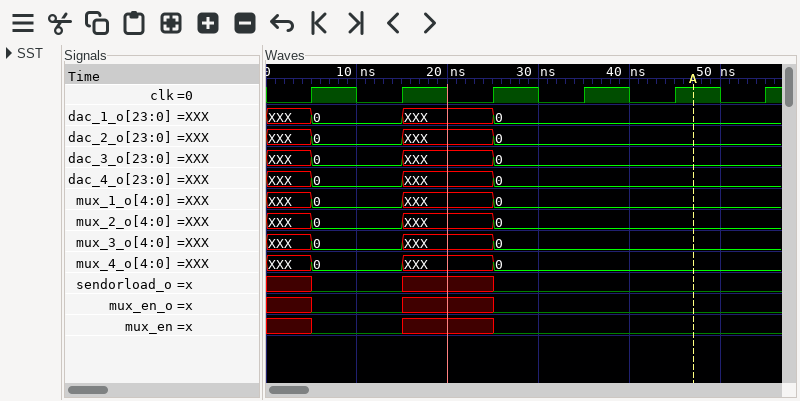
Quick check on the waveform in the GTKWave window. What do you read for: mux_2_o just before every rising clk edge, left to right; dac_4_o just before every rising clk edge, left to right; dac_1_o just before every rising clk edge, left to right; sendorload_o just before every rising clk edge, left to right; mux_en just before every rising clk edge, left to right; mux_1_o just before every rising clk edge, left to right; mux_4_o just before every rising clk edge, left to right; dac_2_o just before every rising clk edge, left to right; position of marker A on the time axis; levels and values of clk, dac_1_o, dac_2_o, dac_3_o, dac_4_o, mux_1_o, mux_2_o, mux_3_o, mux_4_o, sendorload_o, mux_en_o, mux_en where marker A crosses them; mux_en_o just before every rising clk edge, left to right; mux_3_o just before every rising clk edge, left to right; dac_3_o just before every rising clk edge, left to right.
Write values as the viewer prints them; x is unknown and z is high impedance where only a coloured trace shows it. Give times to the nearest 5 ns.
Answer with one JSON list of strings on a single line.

["XXX, 0, XXX, 0, 0, 0", "XXX, 0, XXX, 0, 0, 0", "XXX, 0, XXX, 0, 0, 0", "x 0 x 0 0 0", "x 0 x 0 0 0", "XXX, 0, XXX, 0, 0, 0", "XXX, 0, XXX, 0, 0, 0", "XXX, 0, XXX, 0, 0, 0", "45 ns", "clk=1, dac_1_o=0, dac_2_o=0, dac_3_o=0, dac_4_o=0, mux_1_o=0, mux_2_o=0, mux_3_o=0, mux_4_o=0, sendorload_o=0, mux_en_o=0, mux_en=0", "x 0 x 0 0 0", "XXX, 0, XXX, 0, 0, 0", "XXX, 0, XXX, 0, 0, 0"]
